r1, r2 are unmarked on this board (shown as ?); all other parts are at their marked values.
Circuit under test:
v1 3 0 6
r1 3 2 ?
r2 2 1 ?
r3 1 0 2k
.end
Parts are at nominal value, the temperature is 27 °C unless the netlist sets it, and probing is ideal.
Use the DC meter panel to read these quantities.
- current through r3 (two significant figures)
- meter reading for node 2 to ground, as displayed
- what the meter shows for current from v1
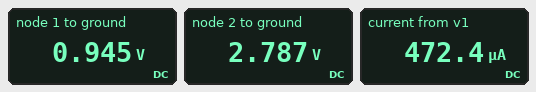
470 µA
2.787 V
472.4 µA
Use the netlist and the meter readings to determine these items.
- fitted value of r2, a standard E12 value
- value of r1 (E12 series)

3.9 kΩ
6.8 kΩ
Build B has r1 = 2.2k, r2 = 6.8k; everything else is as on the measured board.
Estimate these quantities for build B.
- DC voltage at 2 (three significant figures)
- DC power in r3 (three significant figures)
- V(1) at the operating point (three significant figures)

4.80 V
595 µW
1.09 V
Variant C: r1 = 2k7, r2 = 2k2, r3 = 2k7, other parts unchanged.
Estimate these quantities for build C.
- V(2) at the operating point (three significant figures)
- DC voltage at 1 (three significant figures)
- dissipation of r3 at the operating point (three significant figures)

3.87 V
2.13 V
1.68 mW
